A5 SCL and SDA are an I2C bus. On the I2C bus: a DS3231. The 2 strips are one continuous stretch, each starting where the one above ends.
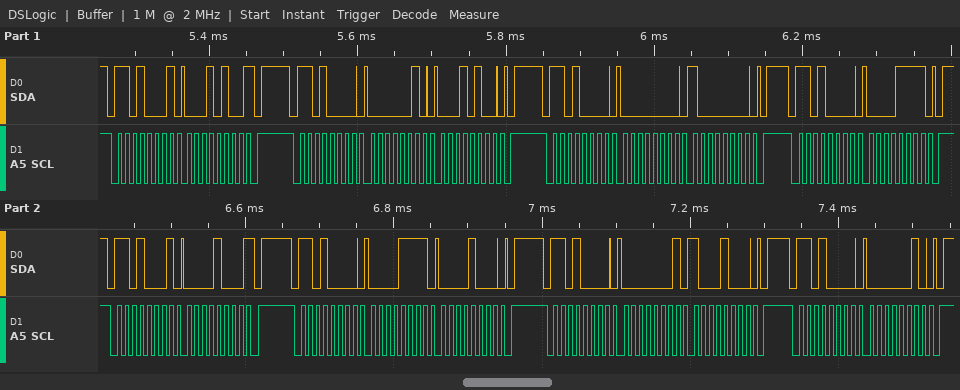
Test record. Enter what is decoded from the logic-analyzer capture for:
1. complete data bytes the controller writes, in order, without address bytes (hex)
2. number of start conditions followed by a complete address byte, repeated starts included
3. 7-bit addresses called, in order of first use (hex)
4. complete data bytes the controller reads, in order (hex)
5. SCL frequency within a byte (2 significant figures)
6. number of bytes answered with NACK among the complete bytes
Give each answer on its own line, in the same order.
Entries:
02 14 00 80 0F 0F 08 01 88 02
8
0x68
14 08
100 kHz
2
